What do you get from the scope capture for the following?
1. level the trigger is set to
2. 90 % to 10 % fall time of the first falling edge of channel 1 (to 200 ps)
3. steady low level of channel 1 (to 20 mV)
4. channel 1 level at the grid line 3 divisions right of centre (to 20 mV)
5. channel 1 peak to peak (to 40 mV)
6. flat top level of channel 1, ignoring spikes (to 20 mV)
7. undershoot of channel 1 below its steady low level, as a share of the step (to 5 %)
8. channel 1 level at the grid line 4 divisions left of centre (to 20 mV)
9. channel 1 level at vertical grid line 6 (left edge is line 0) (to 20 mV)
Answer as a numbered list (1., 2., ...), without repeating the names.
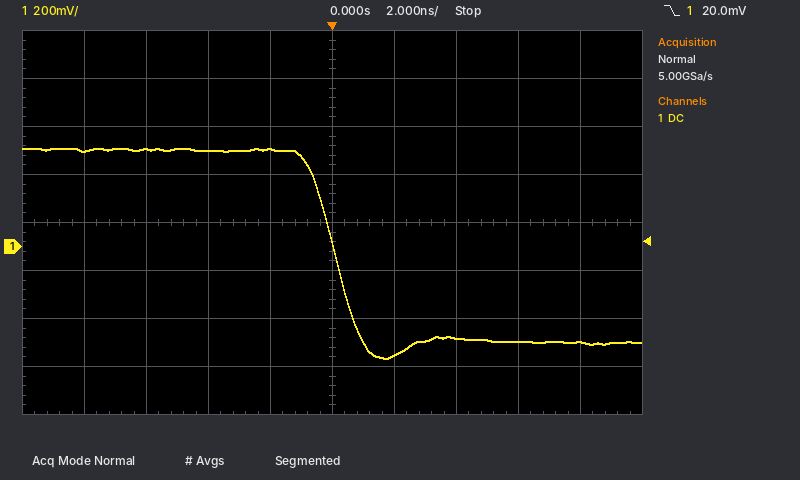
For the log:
1. 20.0 mV
2. 1.4 ns
3. -400 mV
4. -400 mV
5. 880 mV
6. 400 mV
7. 10 %
8. 400 mV
9. -460 mV
